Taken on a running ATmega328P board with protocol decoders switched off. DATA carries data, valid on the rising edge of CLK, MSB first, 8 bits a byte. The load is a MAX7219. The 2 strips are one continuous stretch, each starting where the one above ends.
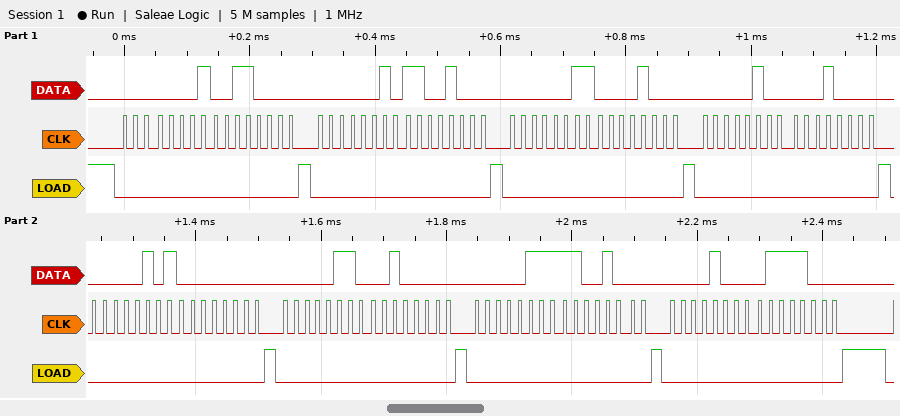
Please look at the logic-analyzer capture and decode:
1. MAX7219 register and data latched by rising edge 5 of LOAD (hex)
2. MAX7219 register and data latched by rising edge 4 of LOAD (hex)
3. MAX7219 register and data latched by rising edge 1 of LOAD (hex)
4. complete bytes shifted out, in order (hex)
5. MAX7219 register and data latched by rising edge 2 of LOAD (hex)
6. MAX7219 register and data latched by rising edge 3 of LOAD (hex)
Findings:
register 0x5, data 0x00
register 0x4, data 0x10
register 0x1, data 0x30
01 30 02 C8 03 08 04 10 05 00 06 20 07 C8 08 78
register 0x2, data 0xC8
register 0x3, data 0x08
